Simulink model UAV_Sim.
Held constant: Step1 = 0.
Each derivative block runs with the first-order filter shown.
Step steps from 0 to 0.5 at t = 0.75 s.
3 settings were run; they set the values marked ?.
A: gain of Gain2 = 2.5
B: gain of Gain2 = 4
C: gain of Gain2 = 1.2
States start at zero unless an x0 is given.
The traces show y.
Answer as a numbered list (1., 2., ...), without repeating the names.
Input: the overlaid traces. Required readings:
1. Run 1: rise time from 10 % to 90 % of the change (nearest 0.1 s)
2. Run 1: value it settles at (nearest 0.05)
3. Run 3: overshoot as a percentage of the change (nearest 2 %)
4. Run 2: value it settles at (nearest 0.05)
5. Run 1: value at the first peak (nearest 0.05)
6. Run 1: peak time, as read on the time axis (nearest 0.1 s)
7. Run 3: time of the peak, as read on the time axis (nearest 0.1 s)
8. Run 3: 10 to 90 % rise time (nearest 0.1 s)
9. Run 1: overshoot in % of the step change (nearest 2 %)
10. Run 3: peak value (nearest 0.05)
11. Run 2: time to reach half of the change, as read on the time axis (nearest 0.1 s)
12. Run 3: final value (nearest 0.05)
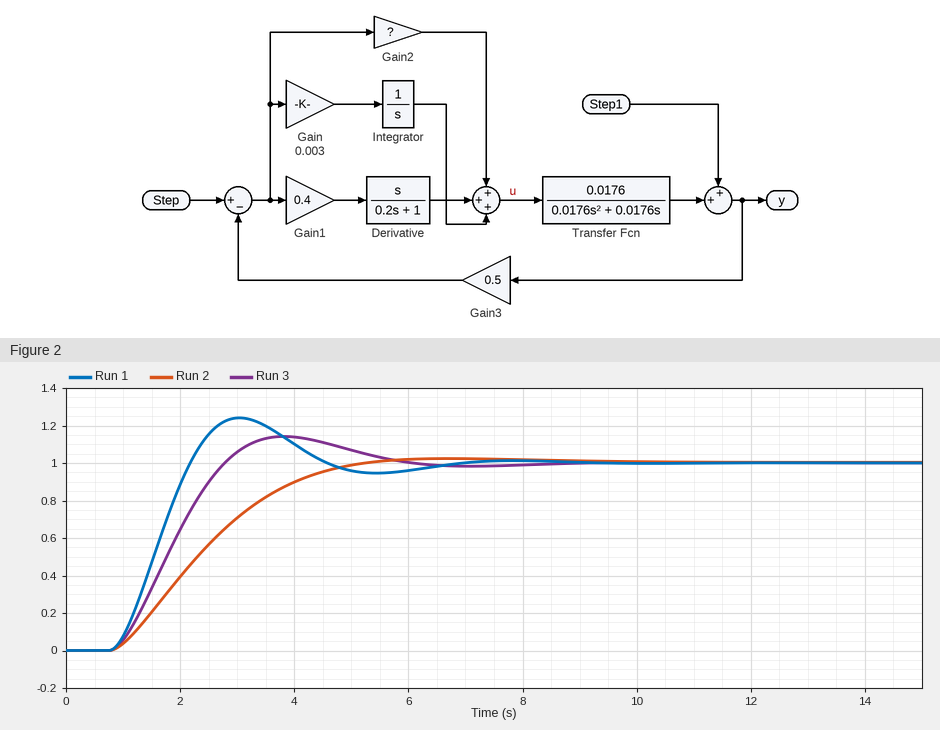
1. 1.0 s
2. 1.00
3. 14 %
4. 1.00
5. 1.25
6. 3.0 s
7. 3.8 s
8. 1.4 s
9. 24 %
10. 1.15
11. 2.3 s
12. 1.00
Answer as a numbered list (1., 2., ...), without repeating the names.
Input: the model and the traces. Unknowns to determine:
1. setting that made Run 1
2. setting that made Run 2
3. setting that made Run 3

1. B
2. C
3. A
